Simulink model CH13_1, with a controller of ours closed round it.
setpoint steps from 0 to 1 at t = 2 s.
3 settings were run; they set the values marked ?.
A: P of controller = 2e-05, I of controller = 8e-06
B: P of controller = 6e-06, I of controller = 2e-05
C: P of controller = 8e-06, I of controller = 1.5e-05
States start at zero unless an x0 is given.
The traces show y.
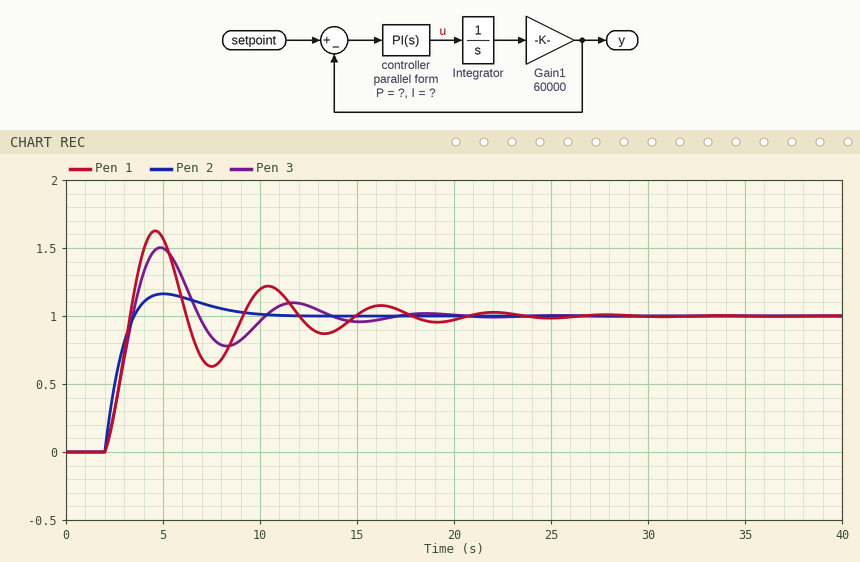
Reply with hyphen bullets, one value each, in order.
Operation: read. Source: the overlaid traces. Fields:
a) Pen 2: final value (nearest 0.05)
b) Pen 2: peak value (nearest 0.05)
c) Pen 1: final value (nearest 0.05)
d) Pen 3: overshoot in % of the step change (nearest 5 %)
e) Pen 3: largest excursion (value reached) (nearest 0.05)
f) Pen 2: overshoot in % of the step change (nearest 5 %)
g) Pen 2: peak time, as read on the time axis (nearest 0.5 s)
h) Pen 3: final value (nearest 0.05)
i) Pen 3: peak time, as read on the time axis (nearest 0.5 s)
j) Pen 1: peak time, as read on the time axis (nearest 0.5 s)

- 1.00
- 1.15
- 1.00
- 50 %
- 1.50
- 15 %
- 5.0 s
- 1.00
- 5.0 s
- 4.5 s
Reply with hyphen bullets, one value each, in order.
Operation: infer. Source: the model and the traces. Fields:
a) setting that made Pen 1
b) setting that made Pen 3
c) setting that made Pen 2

- B
- C
- A
